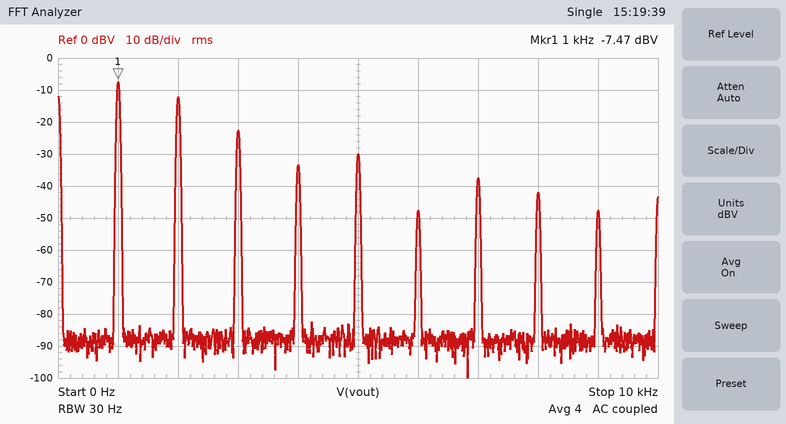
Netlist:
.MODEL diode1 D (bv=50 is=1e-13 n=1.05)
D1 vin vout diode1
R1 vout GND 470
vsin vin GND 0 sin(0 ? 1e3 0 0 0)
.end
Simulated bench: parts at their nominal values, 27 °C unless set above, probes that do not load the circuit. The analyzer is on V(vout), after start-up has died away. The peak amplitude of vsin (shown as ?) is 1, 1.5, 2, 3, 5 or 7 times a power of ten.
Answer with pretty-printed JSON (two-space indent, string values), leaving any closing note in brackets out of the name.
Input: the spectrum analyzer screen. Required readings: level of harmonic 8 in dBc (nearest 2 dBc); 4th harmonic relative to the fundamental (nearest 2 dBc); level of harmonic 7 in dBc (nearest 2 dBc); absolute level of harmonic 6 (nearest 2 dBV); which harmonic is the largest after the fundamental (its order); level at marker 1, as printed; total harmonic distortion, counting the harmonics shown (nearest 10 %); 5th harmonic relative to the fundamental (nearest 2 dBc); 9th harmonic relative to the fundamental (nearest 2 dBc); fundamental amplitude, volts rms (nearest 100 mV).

{
  "level of harmonic 8 in dBc": "-34 dBc",
  "4th harmonic relative to the fundamental": "-26 dBc",
  "level of harmonic 7 in dBc": "-30 dBc",
  "absolute level of harmonic 6": "-48 dBV",
  "which harmonic is the largest after the fundamental": "2",
  "level at marker 1, as printed": "-7.47 dBV",
  "total harmonic distortion, counting the harmonics shown": "60 %",
  "5th harmonic relative to the fundamental": "-22 dBc",
  "9th harmonic relative to the fundamental": "-40 dBc",
  "fundamental amplitude, volts rms": "400 mV"
}
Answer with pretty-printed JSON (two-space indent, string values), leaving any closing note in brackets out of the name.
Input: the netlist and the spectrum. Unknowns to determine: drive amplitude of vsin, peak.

{
  "drive amplitude of vsin, peak": "2 V"
}
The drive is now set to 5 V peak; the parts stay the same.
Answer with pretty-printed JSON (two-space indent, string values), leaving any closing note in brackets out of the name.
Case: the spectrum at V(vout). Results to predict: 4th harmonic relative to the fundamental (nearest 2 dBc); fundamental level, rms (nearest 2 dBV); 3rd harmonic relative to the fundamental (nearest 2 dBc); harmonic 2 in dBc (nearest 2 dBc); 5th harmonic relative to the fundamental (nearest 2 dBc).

{
  "4th harmonic relative to the fundamental": "-22 dBc",
  "fundamental level, rms": "4 dBV",
  "3rd harmonic relative to the fundamental": "-24 dBc",
  "harmonic 2 in dBc": "-6 dBc",
  "5th harmonic relative to the fundamental": "-30 dBc"
}
